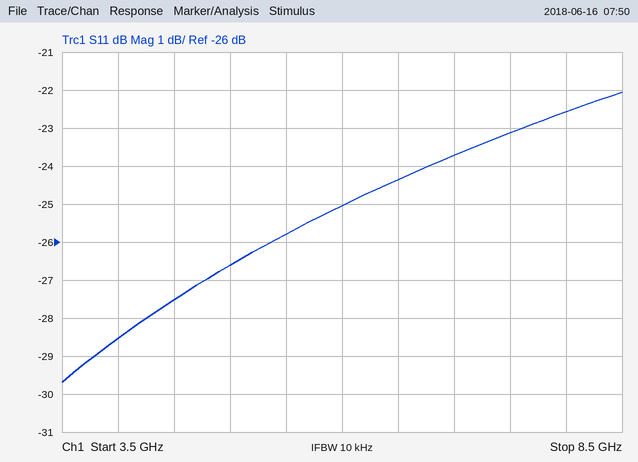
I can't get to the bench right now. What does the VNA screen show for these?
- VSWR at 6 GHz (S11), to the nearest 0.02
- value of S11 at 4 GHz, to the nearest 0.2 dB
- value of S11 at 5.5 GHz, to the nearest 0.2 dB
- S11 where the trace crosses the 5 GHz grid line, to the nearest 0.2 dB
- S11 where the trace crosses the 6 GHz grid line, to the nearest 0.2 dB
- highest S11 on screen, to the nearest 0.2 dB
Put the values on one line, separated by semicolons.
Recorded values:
1.12; -28.6 dB; -25.8 dB; -26.6 dB; -25.0 dB; -22.0 dB
